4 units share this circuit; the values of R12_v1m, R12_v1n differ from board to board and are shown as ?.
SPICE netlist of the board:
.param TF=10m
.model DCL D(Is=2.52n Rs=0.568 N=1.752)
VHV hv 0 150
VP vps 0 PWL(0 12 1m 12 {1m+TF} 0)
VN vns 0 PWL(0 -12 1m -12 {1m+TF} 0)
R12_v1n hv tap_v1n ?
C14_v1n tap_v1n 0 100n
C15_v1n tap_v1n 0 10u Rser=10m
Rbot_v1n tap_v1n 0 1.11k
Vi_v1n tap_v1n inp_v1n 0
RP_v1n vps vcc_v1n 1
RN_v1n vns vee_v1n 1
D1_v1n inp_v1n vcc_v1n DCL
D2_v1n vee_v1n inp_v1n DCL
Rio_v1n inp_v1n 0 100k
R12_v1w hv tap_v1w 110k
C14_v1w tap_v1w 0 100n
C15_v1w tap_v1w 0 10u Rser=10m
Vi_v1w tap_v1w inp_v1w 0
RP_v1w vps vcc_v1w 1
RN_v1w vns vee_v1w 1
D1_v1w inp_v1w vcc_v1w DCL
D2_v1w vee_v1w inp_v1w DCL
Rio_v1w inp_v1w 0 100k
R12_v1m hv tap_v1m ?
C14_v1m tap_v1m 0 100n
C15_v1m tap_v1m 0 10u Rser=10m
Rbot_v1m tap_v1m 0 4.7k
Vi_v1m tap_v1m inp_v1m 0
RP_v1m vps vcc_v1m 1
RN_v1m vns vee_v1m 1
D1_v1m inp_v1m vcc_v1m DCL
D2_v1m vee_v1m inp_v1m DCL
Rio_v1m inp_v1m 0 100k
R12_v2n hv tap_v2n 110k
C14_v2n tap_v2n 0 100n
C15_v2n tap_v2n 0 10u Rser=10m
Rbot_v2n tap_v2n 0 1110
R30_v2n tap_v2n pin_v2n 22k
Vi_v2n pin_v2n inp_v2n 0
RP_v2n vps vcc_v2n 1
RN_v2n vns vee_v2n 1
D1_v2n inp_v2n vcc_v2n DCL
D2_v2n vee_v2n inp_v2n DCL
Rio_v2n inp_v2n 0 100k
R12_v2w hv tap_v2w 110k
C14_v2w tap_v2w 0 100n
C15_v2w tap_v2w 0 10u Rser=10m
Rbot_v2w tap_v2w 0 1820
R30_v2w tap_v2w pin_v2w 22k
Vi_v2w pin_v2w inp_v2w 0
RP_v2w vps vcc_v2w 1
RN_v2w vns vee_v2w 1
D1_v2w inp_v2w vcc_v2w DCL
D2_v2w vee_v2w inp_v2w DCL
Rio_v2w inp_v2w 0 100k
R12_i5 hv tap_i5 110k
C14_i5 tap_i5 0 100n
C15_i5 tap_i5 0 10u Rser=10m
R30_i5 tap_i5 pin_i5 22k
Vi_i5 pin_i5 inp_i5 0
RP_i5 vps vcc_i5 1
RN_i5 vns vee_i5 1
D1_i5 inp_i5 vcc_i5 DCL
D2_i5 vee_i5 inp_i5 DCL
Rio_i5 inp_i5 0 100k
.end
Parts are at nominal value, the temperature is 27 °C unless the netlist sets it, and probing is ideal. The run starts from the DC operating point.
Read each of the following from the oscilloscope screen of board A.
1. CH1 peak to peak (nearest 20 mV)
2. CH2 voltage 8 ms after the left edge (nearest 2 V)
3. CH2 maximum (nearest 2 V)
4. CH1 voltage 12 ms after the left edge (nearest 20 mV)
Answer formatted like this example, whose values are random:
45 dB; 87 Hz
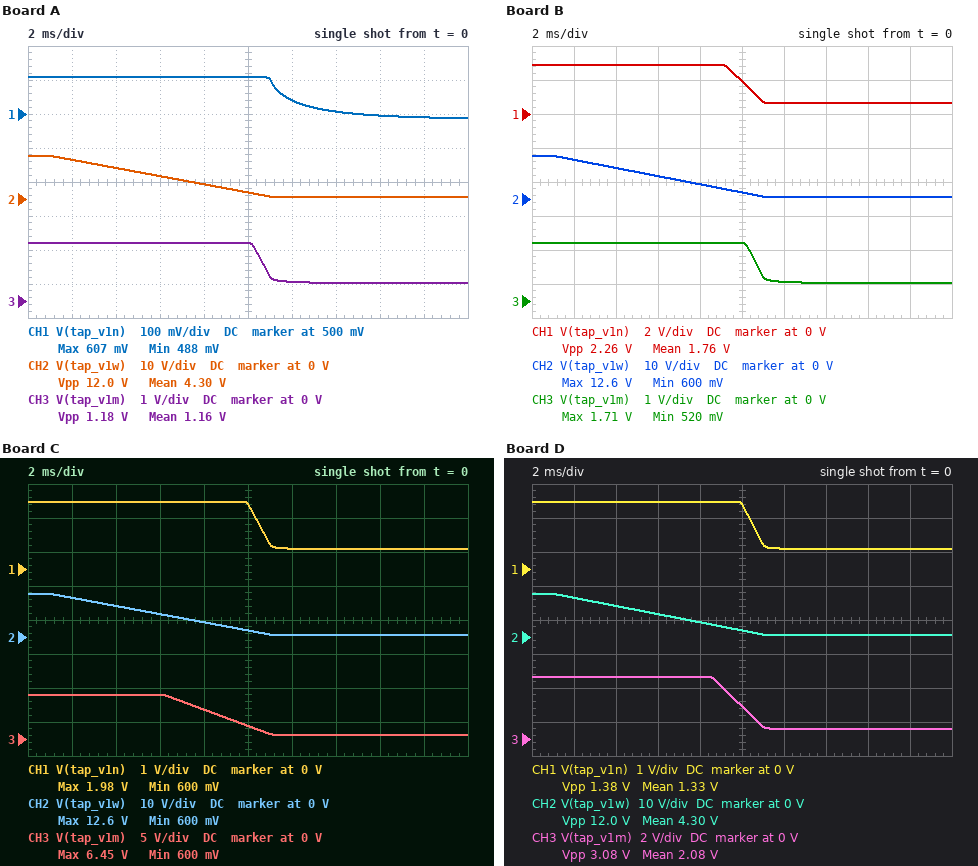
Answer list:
120 mV; 4 V; 12 V; 540 mV
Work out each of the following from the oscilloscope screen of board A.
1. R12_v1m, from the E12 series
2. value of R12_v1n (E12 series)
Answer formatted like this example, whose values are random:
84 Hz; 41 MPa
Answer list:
390 kΩ; 270 kΩ
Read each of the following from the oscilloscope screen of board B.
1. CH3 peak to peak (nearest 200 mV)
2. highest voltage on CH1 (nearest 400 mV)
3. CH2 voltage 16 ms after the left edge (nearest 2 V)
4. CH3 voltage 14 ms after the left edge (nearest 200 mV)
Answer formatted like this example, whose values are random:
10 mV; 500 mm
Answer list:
1.2 V; 2.8 V; 0 V; 600 mV
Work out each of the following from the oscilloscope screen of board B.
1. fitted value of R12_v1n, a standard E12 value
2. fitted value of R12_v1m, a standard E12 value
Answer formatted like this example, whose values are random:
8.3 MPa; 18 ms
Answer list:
56 kΩ; 390 kΩ
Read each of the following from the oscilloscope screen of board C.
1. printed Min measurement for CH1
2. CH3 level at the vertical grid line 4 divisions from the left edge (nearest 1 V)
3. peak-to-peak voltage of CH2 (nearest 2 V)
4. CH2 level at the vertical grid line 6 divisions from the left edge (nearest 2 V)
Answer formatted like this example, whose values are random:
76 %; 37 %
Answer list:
600 mV; 4 V; 12 V; 0 V
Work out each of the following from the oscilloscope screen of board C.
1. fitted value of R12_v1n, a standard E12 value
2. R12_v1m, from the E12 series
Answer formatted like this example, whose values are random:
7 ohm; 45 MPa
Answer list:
82 kΩ; 100 kΩ
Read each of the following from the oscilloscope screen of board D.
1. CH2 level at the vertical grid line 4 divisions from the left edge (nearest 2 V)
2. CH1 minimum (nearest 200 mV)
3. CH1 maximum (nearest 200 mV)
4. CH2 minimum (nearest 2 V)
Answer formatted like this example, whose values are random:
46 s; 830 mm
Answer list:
4 V; 600 mV; 2.0 V; 0 V
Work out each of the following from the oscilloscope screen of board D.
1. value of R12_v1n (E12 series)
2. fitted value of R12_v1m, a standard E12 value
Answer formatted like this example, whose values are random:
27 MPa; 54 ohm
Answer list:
82 kΩ; 180 kΩ
